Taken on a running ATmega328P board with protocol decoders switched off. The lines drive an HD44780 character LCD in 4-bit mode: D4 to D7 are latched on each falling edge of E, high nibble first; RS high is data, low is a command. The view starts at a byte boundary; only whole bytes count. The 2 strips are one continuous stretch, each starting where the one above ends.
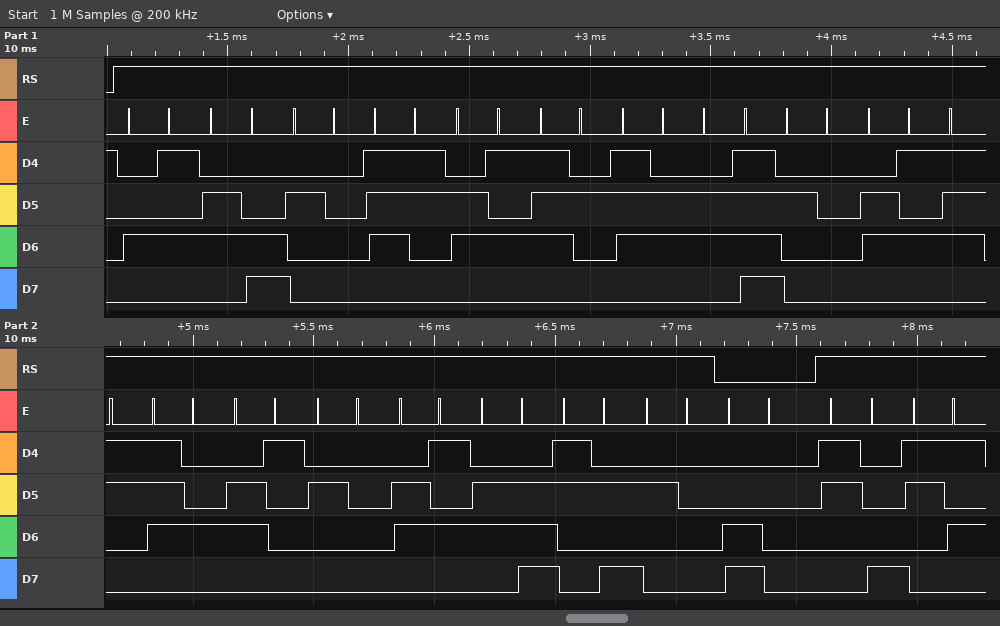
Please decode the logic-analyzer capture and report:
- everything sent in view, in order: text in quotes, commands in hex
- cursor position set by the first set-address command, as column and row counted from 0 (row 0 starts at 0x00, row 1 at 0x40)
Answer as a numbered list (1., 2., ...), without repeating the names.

1. "El servo esta en: " 0xC0 "85"
2. column 0, row 1
